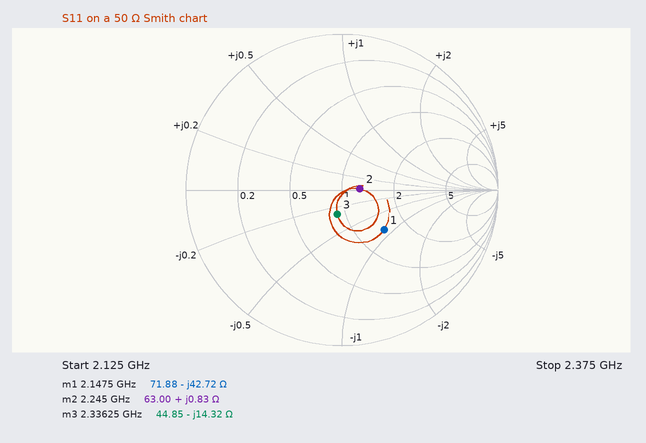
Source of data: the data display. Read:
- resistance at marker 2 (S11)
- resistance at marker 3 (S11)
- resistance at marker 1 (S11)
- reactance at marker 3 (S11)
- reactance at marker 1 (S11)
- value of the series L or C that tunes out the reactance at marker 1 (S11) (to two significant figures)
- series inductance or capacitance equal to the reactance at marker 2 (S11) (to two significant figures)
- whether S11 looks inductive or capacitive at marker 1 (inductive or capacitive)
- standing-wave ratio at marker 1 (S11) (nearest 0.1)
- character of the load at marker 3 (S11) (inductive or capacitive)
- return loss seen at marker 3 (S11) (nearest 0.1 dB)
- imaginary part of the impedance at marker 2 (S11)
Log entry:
63.00 Ω
44.85 Ω
71.88 Ω
-14.32 Ω
-42.72 Ω
3.2 nH
59 pH
capacitive
2.2
capacitive
16.0 dB
+0.83 Ω
